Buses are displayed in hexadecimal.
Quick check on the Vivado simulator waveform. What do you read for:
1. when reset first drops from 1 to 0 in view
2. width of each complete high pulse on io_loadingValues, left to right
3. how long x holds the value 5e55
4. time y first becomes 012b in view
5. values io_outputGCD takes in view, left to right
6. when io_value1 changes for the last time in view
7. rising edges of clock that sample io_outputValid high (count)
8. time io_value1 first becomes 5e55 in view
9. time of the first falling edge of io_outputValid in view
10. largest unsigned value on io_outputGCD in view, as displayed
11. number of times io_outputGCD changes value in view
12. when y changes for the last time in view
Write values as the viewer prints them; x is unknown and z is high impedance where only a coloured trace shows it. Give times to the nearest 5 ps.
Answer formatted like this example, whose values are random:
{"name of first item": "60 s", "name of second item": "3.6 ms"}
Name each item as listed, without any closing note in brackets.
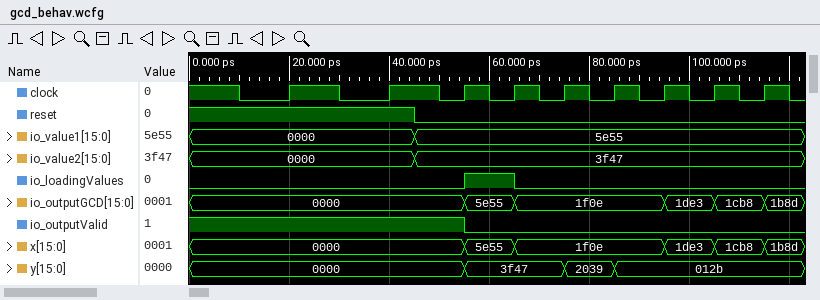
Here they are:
{"when reset first drops from 1 to 0 in view": "45 ps", "width of each complete high pulse on io_loadingValues, left to right": "10 ps", "how long x holds the value 5e55": "10 ps", "time y first becomes 012b in view": "85 ps", "values io_outputGCD takes in view, left to right": "0000, 5e55, 1f0e, 1de3, 1cb8, 1b8d", "when io_value1 changes for the last time in view": "45 ps", "rising edges of clock that sample io_outputValid high": "3", "time io_value1 first becomes 5e55 in view": "45 ps", "time of the first falling edge of io_outputValid in view": "55 ps", "largest unsigned value on io_outputGCD in view, as displayed": "5e55", "number of times io_outputGCD changes value in view": "5", "when y changes for the last time in view": "85 ps"}
